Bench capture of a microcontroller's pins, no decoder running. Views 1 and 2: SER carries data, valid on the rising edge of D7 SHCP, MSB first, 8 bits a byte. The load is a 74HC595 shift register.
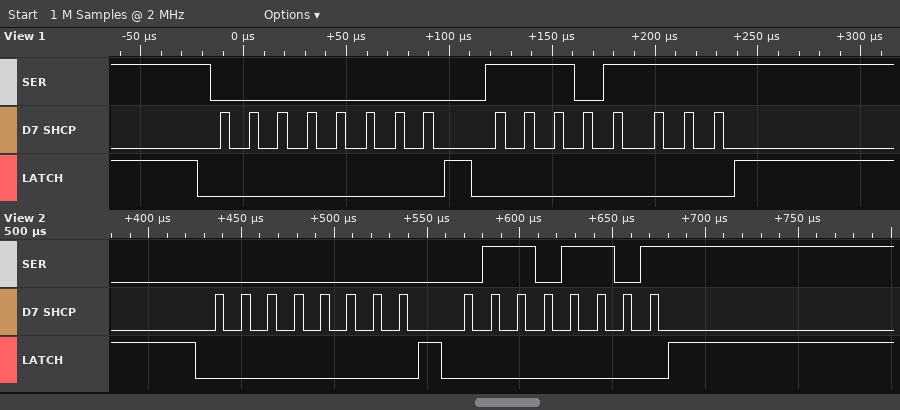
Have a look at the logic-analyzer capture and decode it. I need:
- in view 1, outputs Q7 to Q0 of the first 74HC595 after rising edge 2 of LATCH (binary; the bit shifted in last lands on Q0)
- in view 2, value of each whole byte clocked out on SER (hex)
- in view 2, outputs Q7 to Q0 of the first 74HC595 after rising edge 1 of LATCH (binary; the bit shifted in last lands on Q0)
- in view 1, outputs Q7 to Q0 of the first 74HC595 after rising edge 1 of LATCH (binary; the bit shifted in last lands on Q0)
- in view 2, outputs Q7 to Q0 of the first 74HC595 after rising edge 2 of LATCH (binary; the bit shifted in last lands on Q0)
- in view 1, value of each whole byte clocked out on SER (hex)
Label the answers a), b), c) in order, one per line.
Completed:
a) 11101111
b) 00 6D
c) 00000000
d) 00000000
e) 01101101
f) 00 EF
